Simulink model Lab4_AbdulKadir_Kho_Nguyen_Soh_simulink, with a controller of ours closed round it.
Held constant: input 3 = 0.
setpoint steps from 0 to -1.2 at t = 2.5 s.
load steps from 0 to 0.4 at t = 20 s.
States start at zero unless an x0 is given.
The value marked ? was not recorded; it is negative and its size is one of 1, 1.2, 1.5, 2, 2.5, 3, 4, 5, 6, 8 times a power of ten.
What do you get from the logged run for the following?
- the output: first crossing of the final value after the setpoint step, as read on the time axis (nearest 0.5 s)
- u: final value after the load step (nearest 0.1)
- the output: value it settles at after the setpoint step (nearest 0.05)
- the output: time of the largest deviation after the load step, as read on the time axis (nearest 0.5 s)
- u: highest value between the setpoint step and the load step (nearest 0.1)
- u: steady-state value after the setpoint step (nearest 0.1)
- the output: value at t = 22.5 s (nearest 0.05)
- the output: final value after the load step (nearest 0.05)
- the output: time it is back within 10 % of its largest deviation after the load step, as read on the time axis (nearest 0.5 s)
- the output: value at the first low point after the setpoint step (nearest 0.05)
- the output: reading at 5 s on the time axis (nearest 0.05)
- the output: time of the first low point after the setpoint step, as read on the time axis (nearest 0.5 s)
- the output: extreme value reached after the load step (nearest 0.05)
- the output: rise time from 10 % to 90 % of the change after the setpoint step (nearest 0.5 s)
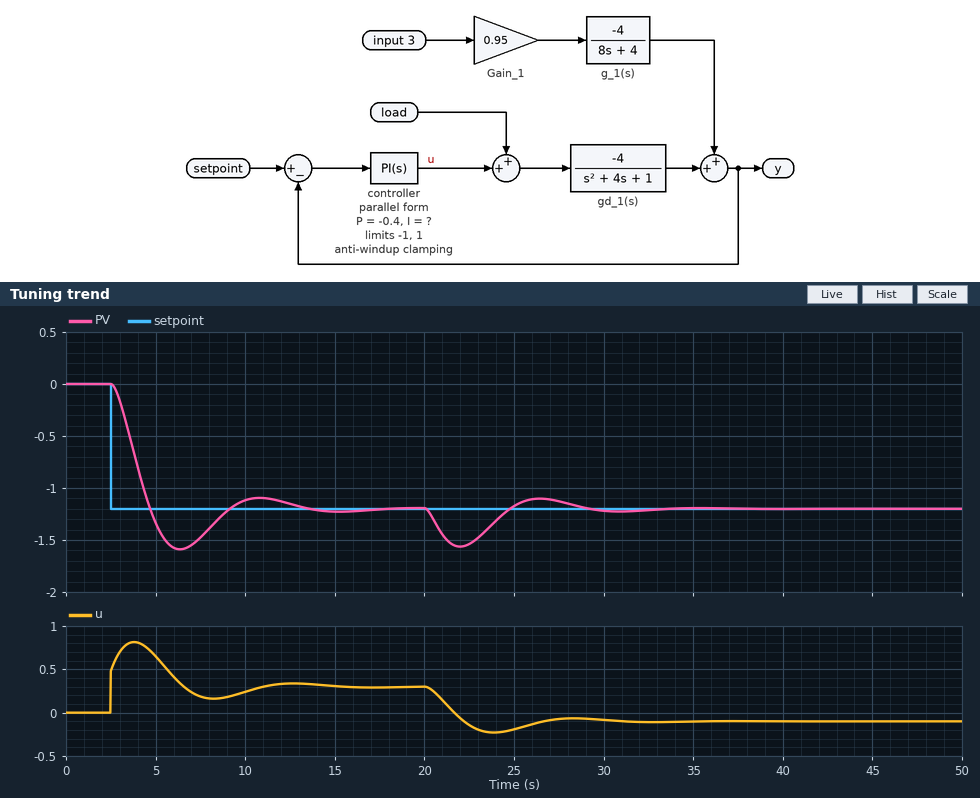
4.5 s
-0.1
-1.20
22.0 s
0.8
0.3
-1.55
-1.20
28.5 s
-1.60
-1.35
6.5 s
-1.55
1.5 s
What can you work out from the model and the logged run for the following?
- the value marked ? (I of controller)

-0.5
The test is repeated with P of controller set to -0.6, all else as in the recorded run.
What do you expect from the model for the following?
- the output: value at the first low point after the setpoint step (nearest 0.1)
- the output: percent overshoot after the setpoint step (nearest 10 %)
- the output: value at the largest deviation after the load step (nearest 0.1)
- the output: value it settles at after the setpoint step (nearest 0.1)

-1.5
20 %
-1.5
-1.2
